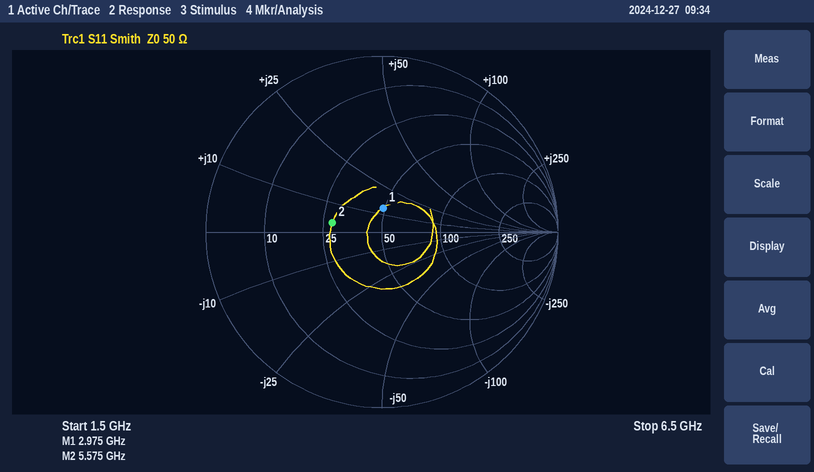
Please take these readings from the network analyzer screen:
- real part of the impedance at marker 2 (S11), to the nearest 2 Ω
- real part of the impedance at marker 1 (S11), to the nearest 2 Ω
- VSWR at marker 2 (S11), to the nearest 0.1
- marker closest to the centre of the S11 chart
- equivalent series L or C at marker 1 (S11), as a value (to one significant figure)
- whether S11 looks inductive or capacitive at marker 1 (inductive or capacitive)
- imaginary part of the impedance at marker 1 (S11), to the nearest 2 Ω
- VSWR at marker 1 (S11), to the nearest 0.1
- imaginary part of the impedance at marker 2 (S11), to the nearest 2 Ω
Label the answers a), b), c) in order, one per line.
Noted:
a) 28 Ω
b) 48 Ω
c) 1.8
d) marker 1
e) 700 pH
f) inductive
g) +14 Ω
h) 1.3
i) +4 Ω
